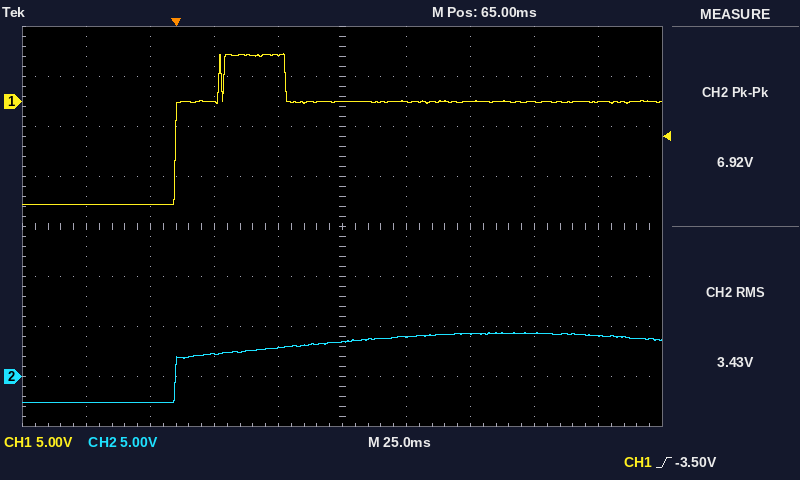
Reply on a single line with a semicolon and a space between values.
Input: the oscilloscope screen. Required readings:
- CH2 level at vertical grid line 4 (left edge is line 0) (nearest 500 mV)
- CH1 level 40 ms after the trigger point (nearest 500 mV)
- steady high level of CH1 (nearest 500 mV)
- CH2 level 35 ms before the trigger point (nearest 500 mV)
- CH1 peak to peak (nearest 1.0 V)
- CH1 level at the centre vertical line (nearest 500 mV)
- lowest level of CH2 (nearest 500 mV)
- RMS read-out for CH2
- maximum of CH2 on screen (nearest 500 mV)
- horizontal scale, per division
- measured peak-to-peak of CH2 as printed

3.0 V; 4.5 V; 0.0 V; -2.5 V; 15.0 V; 0.0 V; -2.5 V; 3.43 V; 4.5 V; 25 ms; 6.92 V
